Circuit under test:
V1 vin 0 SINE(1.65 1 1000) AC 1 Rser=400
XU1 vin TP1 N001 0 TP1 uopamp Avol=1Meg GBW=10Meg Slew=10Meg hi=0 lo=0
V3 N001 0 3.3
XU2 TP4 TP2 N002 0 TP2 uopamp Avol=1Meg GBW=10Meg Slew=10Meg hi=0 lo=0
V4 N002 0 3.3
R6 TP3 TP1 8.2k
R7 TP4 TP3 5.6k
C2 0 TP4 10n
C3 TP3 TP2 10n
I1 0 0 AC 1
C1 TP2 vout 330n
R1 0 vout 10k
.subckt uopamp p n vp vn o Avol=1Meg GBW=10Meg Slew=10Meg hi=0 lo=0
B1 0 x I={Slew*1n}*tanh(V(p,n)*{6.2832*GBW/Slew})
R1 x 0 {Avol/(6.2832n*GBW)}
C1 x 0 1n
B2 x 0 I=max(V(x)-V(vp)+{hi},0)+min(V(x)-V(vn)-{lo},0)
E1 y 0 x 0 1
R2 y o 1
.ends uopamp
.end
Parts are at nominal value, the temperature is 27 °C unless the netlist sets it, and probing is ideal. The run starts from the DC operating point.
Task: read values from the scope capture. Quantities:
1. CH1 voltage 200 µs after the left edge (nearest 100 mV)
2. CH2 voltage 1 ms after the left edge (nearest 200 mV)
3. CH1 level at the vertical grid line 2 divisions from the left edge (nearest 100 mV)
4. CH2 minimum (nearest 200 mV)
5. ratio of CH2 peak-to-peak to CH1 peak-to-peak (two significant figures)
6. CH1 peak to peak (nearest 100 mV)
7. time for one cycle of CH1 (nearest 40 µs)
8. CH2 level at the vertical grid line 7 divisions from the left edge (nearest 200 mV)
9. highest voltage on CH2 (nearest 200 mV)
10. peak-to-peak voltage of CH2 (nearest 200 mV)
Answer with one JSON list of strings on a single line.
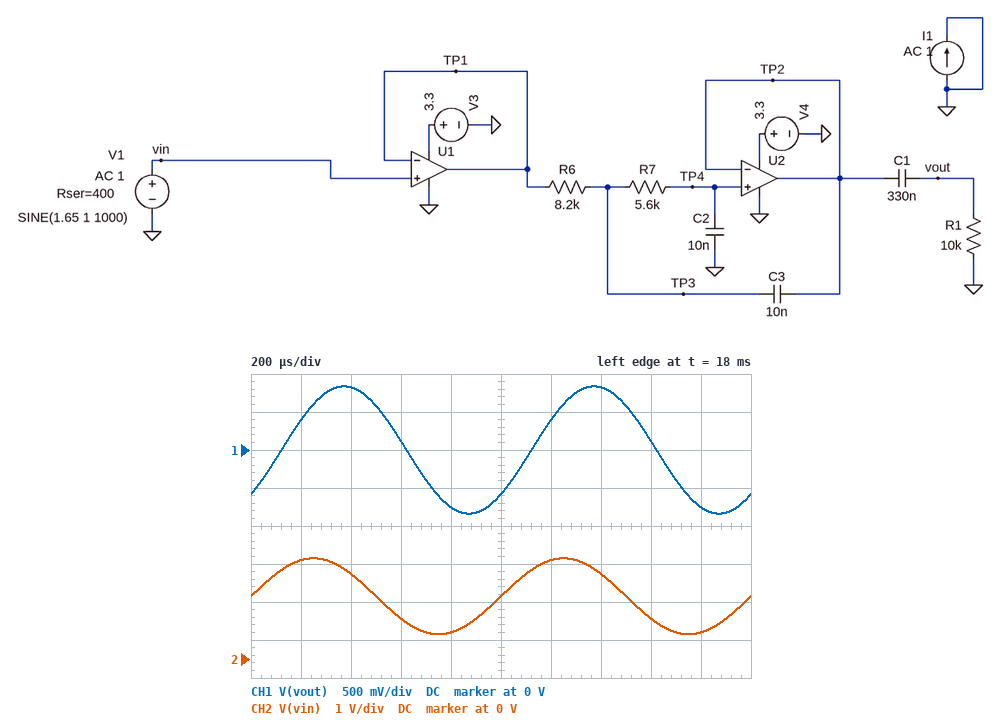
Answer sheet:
["400 mV", "1.6 V", "800 mV", "600 mV", "1.2", "1.7 V", "1.00 ms", "2.2 V", "2.6 V", "2.0 V"]
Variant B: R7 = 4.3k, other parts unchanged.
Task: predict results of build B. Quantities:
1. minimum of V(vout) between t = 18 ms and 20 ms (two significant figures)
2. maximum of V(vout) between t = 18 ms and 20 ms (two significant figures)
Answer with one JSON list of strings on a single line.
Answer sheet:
["-860 mV", "860 mV"]
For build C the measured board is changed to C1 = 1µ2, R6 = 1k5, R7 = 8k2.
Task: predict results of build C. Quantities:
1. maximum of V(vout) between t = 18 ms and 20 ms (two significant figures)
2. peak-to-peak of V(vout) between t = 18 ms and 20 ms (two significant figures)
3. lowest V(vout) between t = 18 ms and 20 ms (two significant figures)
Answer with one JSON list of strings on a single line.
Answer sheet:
["880 mV", "1.8 V", "-890 mV"]
